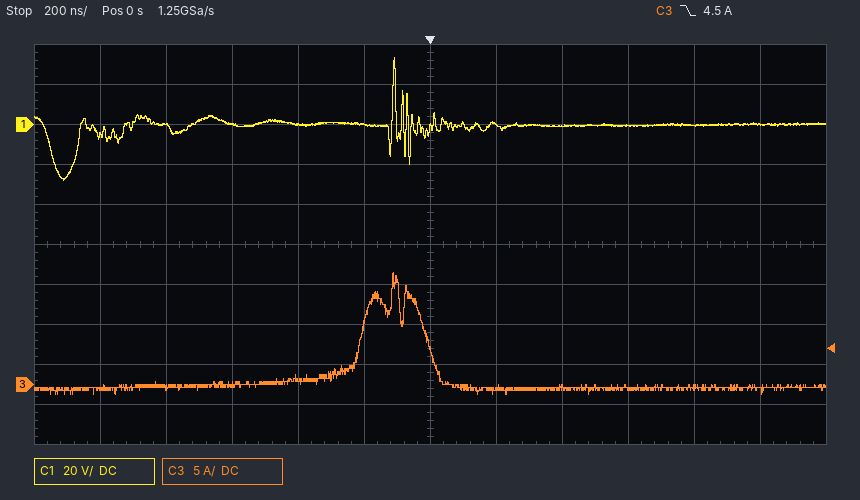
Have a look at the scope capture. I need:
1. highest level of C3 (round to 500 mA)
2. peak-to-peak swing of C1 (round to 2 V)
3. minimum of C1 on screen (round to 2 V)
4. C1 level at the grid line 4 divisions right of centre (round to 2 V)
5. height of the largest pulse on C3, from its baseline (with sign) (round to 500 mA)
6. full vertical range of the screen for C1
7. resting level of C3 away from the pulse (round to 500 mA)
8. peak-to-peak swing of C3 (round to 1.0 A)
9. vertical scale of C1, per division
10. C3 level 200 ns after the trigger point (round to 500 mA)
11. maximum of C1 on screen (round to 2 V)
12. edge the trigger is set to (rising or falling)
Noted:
14.0 A
62 V
-28 V
0 V
+14.5 A
200 V
-500 mA
15.0 A
20 V
-500 mA
34 V
falling
